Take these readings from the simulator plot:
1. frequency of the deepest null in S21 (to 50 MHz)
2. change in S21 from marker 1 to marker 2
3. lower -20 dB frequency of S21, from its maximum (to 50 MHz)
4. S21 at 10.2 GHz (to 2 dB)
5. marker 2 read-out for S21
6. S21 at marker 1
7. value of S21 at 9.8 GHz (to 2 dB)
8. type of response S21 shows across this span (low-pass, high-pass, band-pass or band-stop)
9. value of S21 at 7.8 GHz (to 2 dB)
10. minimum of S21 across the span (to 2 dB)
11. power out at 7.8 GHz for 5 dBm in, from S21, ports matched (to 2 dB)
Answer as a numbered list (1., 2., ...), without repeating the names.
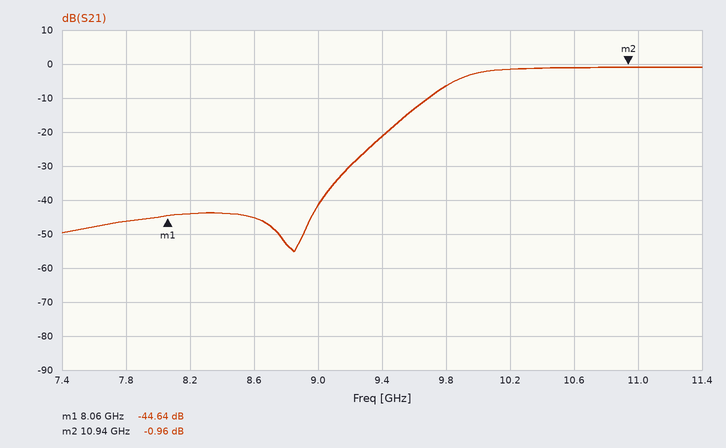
1. 8.85 GHz
2. 43.68 dB
3. 9.40 GHz
4. -2 dB
5. -0.96 dB
6. -44.64 dB
7. -6 dB
8. high-pass
9. -46 dB
10. -56 dB
11. -42 dBm
